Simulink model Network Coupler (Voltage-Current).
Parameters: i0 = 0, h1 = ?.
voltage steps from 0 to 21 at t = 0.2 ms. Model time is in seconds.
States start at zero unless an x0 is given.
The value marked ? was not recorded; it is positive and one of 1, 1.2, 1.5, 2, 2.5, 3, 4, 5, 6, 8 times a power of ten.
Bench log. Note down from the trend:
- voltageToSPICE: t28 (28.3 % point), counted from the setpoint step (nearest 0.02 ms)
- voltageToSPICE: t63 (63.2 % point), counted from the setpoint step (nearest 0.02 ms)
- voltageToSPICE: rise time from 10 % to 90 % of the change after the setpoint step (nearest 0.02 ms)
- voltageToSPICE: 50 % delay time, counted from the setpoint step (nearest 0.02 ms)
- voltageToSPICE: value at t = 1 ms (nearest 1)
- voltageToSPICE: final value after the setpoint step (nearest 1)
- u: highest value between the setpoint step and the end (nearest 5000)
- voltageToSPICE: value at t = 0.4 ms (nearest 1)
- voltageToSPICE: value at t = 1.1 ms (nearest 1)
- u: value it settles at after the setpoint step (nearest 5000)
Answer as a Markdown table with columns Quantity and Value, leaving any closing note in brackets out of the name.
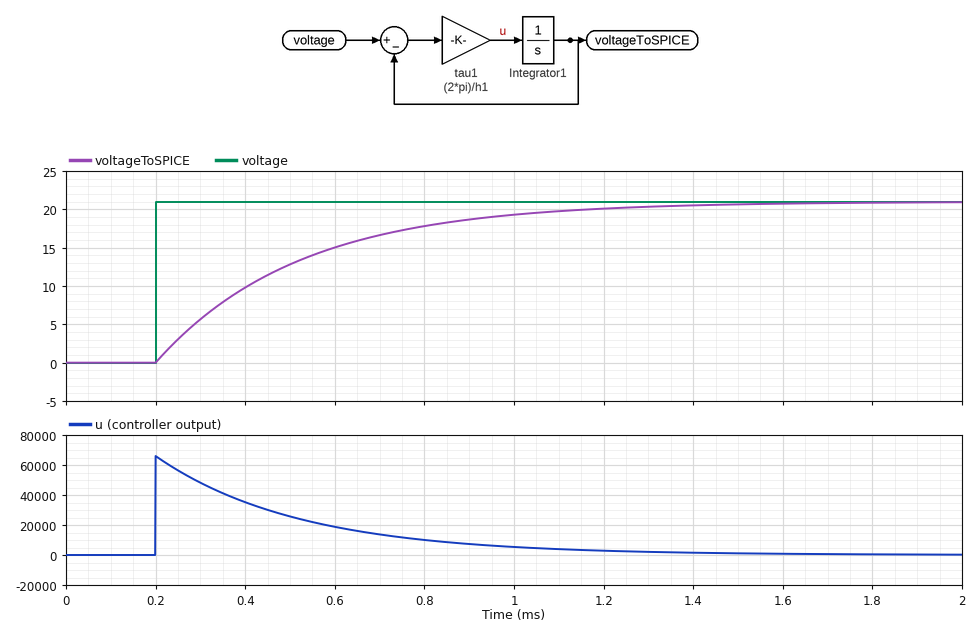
| Quantity | Value |
|---|---|
| voltageToSPICE: t28 (28.3 % point), counted from the setpoint step | 0.10 ms |
| voltageToSPICE: t63 (63.2 % point), counted from the setpoint step | 0.32 ms |
| voltageToSPICE: rise time from 10 % to 90 % of the change after the setpoint step | 0.70 ms |
| voltageToSPICE: 50 % delay time, counted from the setpoint step | 0.22 ms |
| voltageToSPICE: value at t = 1 ms | 19 |
| voltageToSPICE: final value after the setpoint step | 21 |
| u: highest value between the setpoint step and the end | 65000 |
| voltageToSPICE: value at t = 0.4 ms | 10 |
| voltageToSPICE: value at t = 1.1 ms | 20 |
| u: value it settles at after the setpoint step | 0 |
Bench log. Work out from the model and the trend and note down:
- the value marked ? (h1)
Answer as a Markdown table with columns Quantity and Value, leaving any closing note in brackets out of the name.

| Quantity | Value |
|---|---|
| the value marked ? | 0.002 |
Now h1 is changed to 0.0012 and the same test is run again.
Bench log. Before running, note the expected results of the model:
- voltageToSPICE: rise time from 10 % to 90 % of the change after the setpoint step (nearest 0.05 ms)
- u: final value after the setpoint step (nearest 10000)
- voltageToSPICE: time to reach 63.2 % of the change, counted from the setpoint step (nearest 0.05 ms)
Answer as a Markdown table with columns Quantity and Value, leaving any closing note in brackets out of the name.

| Quantity | Value |
|---|---|
| voltageToSPICE: rise time from 10 % to 90 % of the change after the setpoint step | 0.40 ms |
| u: final value after the setpoint step | 0 |
| voltageToSPICE: time to reach 63.2 % of the change, counted from the setpoint step | 0.20 ms |
